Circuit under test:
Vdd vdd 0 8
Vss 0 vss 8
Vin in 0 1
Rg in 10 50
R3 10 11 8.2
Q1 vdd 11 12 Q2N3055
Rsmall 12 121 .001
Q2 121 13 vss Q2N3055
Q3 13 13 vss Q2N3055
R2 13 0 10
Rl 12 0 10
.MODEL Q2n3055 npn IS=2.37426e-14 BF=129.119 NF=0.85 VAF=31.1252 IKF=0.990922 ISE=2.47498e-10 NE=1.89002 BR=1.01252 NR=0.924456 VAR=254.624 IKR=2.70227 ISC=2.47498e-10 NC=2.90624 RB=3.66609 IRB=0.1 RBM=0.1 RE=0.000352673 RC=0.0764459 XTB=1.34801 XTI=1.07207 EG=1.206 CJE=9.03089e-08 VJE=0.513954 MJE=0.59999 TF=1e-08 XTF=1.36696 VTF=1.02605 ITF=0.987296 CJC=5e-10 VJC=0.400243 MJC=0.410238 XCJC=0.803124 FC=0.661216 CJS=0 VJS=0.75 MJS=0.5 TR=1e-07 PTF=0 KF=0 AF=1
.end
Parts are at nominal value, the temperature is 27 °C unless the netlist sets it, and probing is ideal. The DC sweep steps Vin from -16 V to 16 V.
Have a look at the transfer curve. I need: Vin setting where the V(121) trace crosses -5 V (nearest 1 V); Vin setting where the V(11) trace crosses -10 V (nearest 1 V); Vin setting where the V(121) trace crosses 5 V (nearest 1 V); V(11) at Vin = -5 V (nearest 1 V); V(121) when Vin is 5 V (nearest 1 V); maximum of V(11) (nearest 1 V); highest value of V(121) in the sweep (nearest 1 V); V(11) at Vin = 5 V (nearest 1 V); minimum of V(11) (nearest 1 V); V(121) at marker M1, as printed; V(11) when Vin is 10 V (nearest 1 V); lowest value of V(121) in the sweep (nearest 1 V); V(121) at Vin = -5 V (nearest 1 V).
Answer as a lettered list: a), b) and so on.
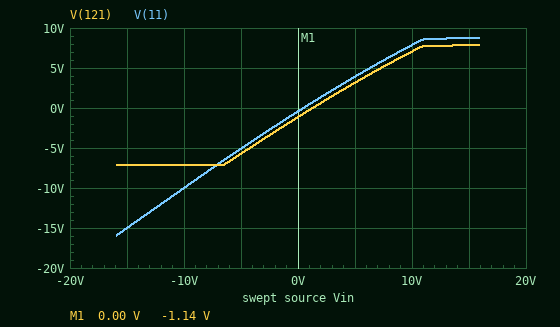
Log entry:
a) -4 V
b) -10 V
c) 7 V
d) -5 V
e) 3 V
f) 9 V
g) 8 V
h) 4 V
i) -16 V
j) -1.14 V
k) 8 V
l) -7 V
m) -6 V
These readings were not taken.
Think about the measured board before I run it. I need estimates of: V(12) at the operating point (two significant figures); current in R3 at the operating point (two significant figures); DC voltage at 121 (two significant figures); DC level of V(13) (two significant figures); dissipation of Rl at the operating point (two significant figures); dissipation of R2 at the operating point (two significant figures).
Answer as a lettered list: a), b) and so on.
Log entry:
a) -250 mV
b) 9.1 mA
c) -250 mV
d) -7.3 V
e) 6.3 mW
f) 5.3 W
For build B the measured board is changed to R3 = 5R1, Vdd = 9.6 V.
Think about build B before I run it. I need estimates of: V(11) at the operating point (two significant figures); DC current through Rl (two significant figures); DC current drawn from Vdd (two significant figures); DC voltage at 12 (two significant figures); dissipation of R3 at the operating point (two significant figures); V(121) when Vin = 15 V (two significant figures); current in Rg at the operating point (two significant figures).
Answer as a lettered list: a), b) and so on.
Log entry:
a) 520 mV
b) 20 mA
c) 840 mA
d) -200 mV
e) 390 µW
f) 9.4 V
g) 8.7 mA
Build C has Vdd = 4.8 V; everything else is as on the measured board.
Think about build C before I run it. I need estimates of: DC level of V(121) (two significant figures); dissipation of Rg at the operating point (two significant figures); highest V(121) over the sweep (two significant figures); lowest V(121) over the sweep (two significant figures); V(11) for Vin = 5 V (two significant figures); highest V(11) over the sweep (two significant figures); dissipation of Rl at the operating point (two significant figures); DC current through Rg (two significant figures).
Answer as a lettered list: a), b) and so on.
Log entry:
a) -310 mV
b) 5.1 mW
c) 4.7 V
d) -7.1 V
e) 3.8 V
f) 5.7 V
g) 9.8 mW
h) 10 mA
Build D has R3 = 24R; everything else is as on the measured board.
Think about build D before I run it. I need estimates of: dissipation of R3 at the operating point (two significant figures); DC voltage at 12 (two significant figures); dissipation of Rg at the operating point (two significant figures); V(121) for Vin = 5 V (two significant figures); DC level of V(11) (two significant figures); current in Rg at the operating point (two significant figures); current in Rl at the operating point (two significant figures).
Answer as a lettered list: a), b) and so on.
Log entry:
a) 1.9 mW
b) -370 mV
c) 3.9 mW
d) 2.9 V
e) 350 mV
f) 8.8 mA
g) 37 mA
